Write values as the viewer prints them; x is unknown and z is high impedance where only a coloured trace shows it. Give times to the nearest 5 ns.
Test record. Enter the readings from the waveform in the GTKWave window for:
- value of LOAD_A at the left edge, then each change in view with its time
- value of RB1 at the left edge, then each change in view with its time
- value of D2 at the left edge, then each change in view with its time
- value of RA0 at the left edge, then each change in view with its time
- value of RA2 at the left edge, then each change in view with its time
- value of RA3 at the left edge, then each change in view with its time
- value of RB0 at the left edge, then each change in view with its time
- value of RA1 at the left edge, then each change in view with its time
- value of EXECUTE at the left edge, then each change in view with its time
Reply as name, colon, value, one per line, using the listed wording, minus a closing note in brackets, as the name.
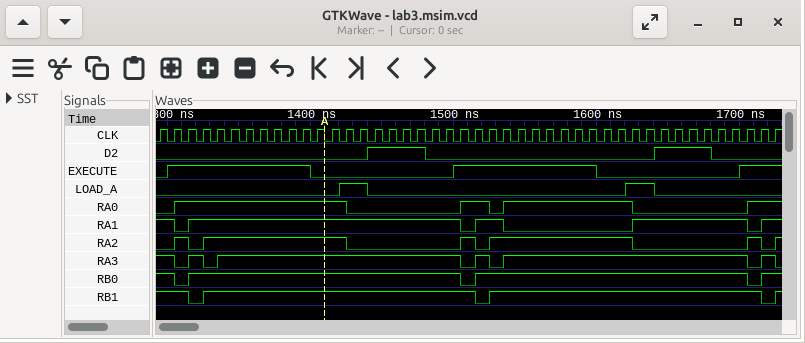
value of LOAD_A at the left edge, then each change in view with its time: 0, 1 at 1420 ns, 0 at 1440 ns, 1 at 1620 ns, 0 at 1640 ns
value of RB1 at the left edge, then each change in view with its time: 1, 0 at 1315 ns, 1 at 1325 ns, 0 at 1515 ns, 1 at 1525 ns, 0 at 1715 ns, 1 at 1725 ns
value of D2 at the left edge, then each change in view with its time: 0, 1 at 1440 ns, 0 at 1480 ns, 1 at 1640 ns, 0 at 1680 ns
value of RA0 at the left edge, then each change in view with its time: 0, 1 at 1305 ns, 0 at 1425 ns, 1 at 1505 ns, 0 at 1525 ns, 1 at 1535 ns, 0 at 1625 ns, 1 at 1705 ns
value of RA2 at the left edge, then each change in view with its time: 0, 1 at 1305 ns, 0 at 1315 ns, 1 at 1325 ns, 0 at 1425 ns, 1 at 1505 ns, 0 at 1515 ns, 1 at 1525 ns, 0 at 1625 ns, 1 at 1705 ns, 0 at 1715 ns, 1 at 1725 ns
value of RA3 at the left edge, then each change in view with its time: 1, 0 at 1305 ns, 1 at 1315 ns, 0 at 1325 ns, 1 at 1335 ns, 0 at 1505 ns, 1 at 1515 ns, 0 at 1525 ns, 1 at 1535 ns, 0 at 1705 ns, 1 at 1715 ns, 0 at 1725 ns
value of RB0 at the left edge, then each change in view with its time: 1, 0 at 1305 ns, 1 at 1315 ns, 0 at 1505 ns, 1 at 1515 ns, 0 at 1705 ns, 1 at 1715 ns
value of RA1 at the left edge, then each change in view with its time: 1, 0 at 1305 ns, 1 at 1315 ns, 0 at 1505 ns, 1 at 1515 ns, 0 at 1535 ns, 1 at 1625 ns, 0 at 1705 ns, 1 at 1715 ns
value of EXECUTE at the left edge, then each change in view with its time: 0, 1 at 1300 ns, 0 at 1400 ns, 1 at 1500 ns, 0 at 1600 ns, 1 at 1700 ns
